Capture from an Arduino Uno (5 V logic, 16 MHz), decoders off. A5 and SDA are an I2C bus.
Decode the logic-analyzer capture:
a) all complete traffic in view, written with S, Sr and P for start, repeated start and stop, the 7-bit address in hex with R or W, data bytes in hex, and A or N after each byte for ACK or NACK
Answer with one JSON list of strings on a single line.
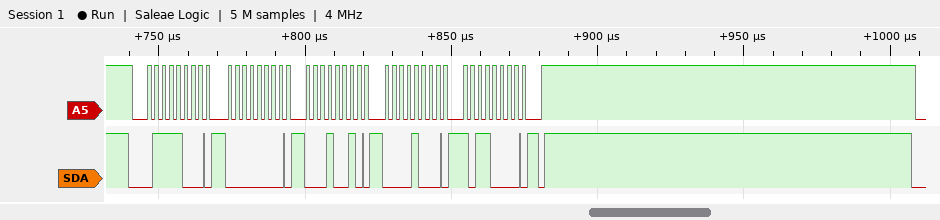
["S 3CW A 00 A 12 A 08 A B0 A P"]
